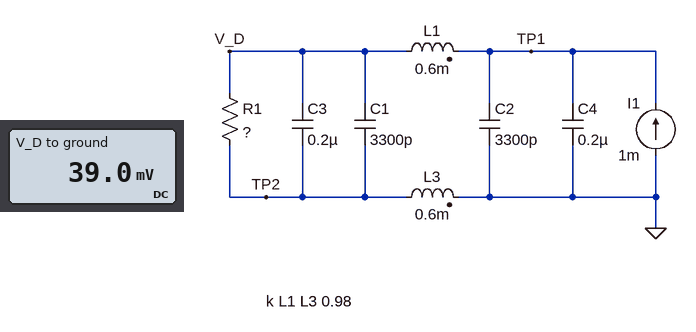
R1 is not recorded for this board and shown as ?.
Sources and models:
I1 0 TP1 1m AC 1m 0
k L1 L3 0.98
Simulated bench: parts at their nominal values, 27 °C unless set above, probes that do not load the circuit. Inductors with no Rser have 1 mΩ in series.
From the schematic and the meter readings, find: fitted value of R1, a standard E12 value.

39 Ω
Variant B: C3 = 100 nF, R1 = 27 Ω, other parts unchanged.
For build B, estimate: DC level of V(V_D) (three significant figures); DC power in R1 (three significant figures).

27.0 mV
27.0 µW
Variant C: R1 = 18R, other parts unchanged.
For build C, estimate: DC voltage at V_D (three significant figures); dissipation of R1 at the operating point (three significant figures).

18.0 mV
18.0 µW
